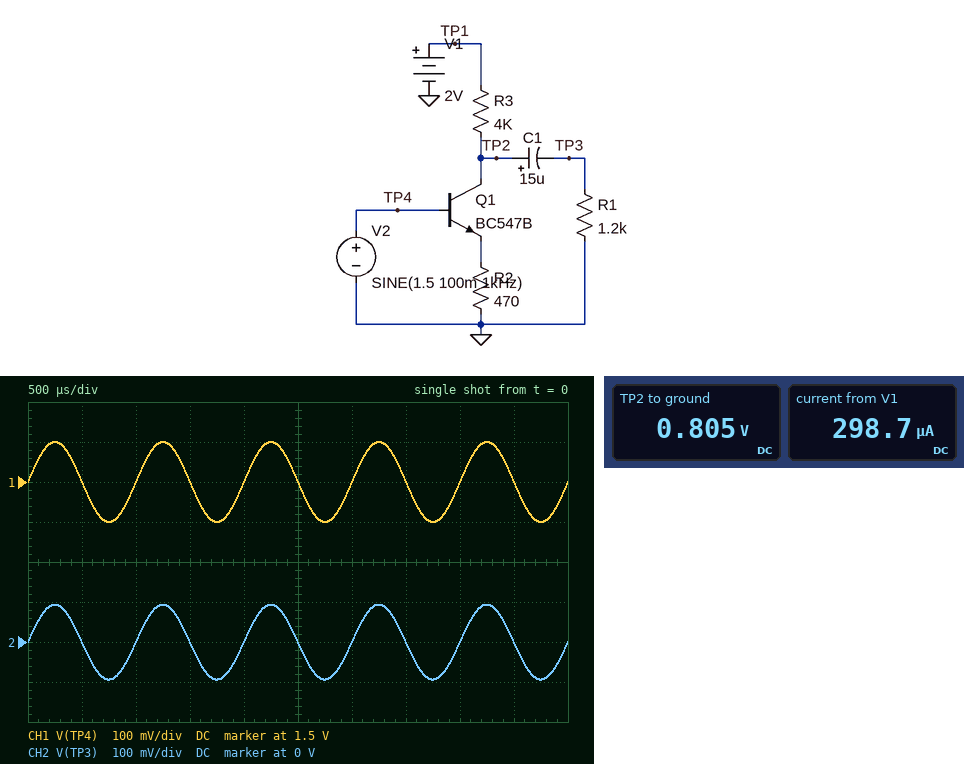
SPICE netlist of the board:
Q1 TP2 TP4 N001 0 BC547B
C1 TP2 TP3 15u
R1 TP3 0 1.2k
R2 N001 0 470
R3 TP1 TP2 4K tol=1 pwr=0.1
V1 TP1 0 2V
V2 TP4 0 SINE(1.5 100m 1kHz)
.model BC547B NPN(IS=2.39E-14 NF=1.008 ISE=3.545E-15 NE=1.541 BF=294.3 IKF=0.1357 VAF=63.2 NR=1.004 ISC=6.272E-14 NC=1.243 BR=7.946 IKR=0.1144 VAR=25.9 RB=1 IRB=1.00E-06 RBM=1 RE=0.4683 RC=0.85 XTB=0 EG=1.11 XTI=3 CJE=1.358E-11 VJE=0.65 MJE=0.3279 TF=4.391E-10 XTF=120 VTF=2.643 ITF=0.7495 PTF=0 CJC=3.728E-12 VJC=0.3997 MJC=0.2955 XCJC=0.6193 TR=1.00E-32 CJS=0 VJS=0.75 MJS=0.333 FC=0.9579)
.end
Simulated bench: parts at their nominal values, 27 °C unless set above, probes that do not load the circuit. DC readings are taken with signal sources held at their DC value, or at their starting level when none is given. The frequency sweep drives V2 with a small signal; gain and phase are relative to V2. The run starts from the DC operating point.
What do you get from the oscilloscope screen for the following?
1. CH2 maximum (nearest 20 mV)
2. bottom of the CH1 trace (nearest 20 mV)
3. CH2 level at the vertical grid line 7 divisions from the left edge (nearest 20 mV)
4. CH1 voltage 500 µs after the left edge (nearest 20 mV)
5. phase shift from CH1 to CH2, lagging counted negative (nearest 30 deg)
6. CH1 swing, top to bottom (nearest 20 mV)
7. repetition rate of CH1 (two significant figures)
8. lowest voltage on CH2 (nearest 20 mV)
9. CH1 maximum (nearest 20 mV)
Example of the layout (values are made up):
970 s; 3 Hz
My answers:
100 mV; 1.40 V; 0 V; 1.50 V; 0 deg; 200 mV; 1.0 kHz; -100 mV; 1.60 V
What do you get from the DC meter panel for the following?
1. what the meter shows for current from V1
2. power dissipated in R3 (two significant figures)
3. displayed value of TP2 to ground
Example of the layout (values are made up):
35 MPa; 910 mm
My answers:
298.7 µA; 360 µW; 0.805 V
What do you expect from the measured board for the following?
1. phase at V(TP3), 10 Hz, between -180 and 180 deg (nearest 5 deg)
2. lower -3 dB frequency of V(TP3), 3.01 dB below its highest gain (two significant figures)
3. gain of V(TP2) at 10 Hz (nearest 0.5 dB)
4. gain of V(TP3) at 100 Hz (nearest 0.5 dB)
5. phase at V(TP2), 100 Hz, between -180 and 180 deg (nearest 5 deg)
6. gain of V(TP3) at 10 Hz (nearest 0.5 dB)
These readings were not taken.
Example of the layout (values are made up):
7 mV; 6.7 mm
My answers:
40 deg; 8.7 Hz; -0.5 dB; -0.5 dB; 0 deg; -3.0 dB
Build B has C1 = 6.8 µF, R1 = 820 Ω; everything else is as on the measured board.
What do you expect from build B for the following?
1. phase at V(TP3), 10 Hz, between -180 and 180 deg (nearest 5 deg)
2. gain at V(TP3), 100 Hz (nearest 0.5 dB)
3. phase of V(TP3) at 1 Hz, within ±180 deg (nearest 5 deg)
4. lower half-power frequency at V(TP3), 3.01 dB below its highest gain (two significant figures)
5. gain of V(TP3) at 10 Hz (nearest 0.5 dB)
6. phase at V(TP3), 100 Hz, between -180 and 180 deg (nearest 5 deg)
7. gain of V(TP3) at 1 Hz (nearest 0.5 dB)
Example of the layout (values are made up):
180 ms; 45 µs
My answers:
70 deg; -1.0 dB; 90 deg; 28 Hz; -10.0 dB; 15 deg; -29.5 dB
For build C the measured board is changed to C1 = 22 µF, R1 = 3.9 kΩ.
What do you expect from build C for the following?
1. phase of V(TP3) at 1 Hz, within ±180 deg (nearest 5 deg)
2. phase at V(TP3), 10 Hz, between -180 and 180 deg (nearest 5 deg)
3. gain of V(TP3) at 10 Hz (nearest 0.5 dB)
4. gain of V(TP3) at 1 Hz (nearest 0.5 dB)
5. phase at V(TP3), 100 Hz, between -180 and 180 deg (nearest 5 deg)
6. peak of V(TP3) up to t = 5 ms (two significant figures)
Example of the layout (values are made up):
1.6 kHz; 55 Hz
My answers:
60 deg; 10 deg; -0.5 dB; -7.0 dB; 0 deg; 95 mV
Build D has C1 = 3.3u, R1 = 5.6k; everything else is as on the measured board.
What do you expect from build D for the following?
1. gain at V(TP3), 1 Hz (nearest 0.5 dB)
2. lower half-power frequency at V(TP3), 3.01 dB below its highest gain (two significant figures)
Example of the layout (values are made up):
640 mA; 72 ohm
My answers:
-19.0 dB; 8.6 Hz
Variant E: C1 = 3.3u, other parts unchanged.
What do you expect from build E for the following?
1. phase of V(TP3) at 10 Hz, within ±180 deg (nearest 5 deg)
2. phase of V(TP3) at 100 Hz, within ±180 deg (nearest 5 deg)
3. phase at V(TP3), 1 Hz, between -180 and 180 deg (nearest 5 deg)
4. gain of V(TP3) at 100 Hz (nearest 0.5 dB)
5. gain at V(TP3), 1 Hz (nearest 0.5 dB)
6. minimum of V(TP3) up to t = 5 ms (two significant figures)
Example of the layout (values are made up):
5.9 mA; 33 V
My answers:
75 deg; 20 deg; 90 deg; -1.0 dB; -32.5 dB; -96 mV
